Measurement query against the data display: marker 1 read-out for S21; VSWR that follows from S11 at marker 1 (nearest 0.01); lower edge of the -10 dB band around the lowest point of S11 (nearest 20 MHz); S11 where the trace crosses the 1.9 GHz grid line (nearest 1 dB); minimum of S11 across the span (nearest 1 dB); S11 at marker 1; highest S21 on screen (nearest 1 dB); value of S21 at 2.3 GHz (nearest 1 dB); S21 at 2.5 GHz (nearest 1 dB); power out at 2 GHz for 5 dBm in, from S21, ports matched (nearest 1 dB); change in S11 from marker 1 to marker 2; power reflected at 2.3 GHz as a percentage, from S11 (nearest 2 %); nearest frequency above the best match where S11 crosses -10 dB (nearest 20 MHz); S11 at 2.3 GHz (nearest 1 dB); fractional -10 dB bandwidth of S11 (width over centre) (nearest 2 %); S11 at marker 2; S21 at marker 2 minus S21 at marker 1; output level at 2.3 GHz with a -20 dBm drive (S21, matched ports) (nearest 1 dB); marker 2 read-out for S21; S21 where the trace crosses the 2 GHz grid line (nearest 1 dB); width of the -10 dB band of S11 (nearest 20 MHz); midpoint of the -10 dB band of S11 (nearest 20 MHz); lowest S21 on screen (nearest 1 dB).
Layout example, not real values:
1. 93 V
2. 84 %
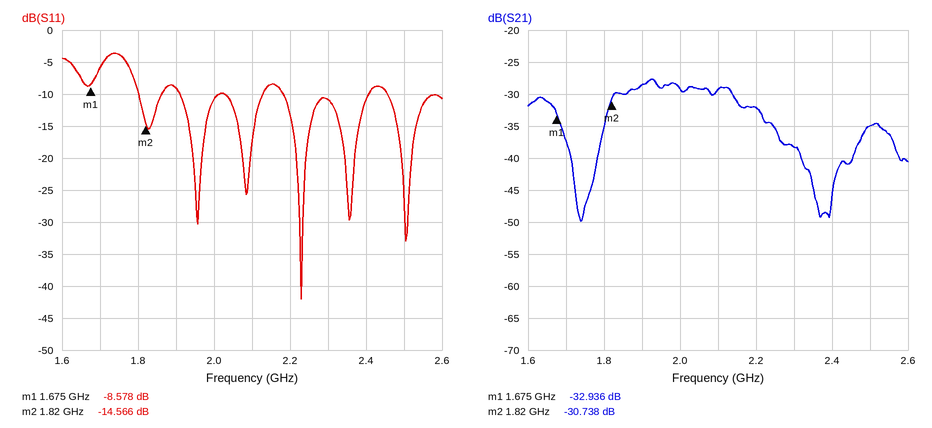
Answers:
1. -32.936 dB
2. 2.19
3. 2.18 GHz
4. -9 dB
5. -42 dB
6. -8.578 dB
7. -28 dB
8. -38 dB
9. -35 dB
10. -24 dBm
11. -5.988 dB
12. 8 %
13. 2.40 GHz
14. -11 dB
15. 10 %
16. -14.566 dB
17. 2.198 dB
18. -58 dBm
19. -30.738 dB
20. -29 dB
21. 220 MHz
22. 2.30 GHz
23. -50 dB
